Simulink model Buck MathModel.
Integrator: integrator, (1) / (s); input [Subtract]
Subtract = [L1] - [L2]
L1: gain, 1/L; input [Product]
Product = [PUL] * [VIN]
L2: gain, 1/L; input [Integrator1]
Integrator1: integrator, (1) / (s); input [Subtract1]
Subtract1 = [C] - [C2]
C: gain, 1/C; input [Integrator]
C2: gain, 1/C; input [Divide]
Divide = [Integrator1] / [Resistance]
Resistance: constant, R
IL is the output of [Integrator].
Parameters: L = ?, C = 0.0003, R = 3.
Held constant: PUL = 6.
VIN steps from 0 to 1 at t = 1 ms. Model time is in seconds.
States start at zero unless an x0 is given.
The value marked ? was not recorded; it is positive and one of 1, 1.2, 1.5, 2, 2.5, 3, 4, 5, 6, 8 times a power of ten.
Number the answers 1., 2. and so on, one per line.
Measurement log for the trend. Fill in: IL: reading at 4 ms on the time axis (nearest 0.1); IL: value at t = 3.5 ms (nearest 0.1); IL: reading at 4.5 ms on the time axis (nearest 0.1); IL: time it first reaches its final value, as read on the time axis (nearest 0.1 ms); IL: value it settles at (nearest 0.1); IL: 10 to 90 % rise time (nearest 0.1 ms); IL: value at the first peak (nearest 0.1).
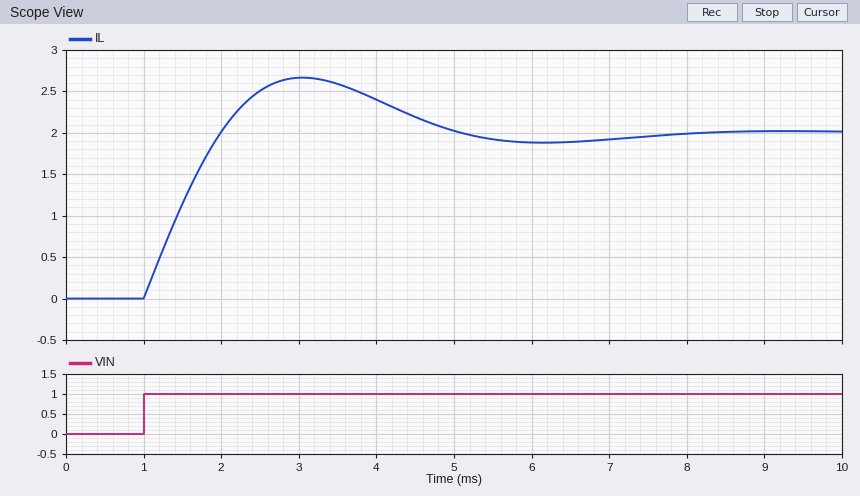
1. 2.4
2. 2.6
3. 2.2
4. 2.0 ms
5. 2.0
6. 0.8 ms
7. 2.7
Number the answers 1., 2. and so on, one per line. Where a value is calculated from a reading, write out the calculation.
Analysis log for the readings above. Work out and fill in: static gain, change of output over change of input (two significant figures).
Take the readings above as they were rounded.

1. (2 - 0) / (1 - 0) = 2.0
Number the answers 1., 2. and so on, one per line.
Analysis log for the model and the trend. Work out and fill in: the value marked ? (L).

1. 0.0025
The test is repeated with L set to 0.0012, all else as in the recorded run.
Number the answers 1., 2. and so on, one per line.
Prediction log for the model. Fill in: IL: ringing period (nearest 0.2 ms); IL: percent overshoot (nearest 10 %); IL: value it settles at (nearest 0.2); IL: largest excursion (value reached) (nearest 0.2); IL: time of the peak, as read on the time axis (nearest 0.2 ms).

1. 4.0 ms
2. 80 %
3. 2.0
4. 3.6
5. 2.2 ms
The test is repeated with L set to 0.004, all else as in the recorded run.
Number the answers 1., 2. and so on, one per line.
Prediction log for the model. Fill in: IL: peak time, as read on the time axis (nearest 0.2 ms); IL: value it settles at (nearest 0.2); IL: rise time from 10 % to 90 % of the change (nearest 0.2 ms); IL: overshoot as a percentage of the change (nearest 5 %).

1. 4.0 ms
2. 2.0
3. 1.4 ms
4. 15 %
